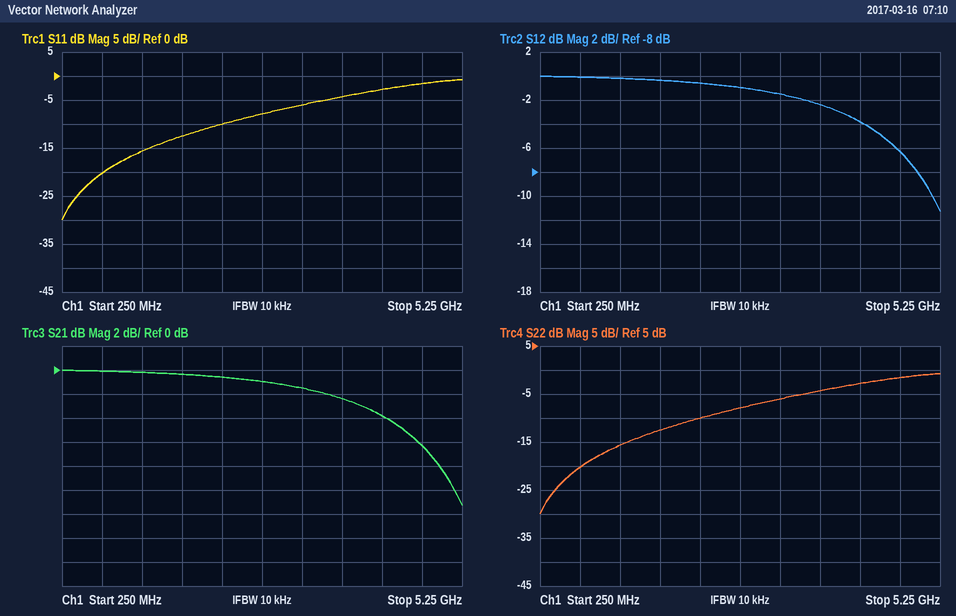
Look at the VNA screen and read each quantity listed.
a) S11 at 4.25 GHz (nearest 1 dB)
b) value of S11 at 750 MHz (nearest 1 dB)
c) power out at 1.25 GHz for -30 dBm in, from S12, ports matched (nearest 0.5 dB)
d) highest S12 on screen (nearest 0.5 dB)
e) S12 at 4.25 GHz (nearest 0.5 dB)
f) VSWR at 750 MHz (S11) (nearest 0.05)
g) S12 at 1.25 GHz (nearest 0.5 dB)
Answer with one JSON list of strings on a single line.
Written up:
["-3 dB", "-20 dB", "-30.0 dBm", "0.0 dB", "-4.0 dB", "1.20", "0.0 dB"]
